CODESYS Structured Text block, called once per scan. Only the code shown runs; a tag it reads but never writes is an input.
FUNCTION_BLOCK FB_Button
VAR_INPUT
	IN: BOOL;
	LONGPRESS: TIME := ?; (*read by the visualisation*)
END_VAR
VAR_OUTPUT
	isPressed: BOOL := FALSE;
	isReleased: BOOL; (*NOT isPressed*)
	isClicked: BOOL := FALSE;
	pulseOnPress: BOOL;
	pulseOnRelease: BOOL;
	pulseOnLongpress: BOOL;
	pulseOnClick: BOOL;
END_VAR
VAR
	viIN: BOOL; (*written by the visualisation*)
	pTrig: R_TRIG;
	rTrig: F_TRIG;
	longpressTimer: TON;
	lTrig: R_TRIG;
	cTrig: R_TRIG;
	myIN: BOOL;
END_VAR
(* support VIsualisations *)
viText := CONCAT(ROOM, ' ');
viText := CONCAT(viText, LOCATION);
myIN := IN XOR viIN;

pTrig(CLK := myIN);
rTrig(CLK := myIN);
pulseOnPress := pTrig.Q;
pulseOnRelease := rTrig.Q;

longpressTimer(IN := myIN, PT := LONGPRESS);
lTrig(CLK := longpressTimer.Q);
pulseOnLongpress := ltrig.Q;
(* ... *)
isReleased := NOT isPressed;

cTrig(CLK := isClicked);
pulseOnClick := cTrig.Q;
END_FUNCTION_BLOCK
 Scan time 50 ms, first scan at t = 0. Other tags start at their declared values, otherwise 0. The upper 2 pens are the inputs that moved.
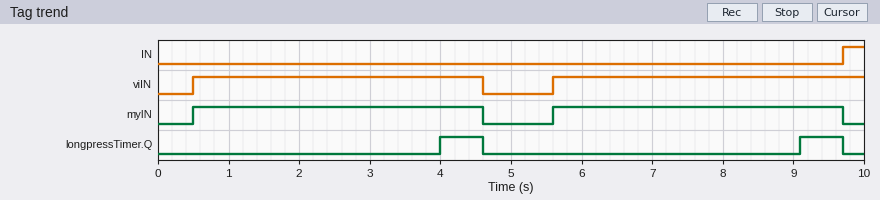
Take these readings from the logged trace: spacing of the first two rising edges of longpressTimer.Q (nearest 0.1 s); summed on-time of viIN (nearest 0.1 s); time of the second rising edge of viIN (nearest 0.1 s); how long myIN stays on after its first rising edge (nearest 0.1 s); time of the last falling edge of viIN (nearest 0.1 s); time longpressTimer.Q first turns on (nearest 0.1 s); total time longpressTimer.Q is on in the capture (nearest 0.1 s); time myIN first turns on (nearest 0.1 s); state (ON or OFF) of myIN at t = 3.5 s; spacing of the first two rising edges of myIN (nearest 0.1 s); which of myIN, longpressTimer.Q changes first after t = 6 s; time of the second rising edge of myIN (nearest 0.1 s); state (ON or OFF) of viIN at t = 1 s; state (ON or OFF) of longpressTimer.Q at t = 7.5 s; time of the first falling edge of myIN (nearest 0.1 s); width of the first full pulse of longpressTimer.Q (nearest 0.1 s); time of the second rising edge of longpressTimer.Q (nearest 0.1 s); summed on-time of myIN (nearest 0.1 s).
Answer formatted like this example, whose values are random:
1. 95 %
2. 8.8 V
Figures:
1. 5.1 s
2. 8.5 s
3. 5.6 s
4. 4.1 s
5. 4.6 s
6. 4.0 s
7. 1.2 s
8. 0.5 s
9. ON
10. 5.1 s
11. longpressTimer.Q
12. 5.6 s
13. ON
14. OFF
15. 4.6 s
16. 0.6 s
17. 9.1 s
18. 8.2 s
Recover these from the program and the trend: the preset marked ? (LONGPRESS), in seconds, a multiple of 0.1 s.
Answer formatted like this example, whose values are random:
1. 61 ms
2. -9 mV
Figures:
1. 3.5 s
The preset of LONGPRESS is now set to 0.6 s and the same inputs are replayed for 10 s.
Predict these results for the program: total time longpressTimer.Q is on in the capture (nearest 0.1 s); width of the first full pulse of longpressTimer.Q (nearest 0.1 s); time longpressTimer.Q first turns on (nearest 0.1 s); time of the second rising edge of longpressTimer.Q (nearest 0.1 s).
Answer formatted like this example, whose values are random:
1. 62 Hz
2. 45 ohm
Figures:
1. 7.0 s
2. 3.5 s
3. 1.1 s
4. 6.2 s
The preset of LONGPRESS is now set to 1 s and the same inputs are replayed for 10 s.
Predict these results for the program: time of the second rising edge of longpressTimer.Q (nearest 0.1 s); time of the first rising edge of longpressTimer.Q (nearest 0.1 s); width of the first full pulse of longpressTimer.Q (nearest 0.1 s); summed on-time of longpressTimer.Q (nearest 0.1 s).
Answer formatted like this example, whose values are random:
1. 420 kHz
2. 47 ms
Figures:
1. 6.6 s
2. 1.5 s
3. 3.1 s
4. 6.2 s
